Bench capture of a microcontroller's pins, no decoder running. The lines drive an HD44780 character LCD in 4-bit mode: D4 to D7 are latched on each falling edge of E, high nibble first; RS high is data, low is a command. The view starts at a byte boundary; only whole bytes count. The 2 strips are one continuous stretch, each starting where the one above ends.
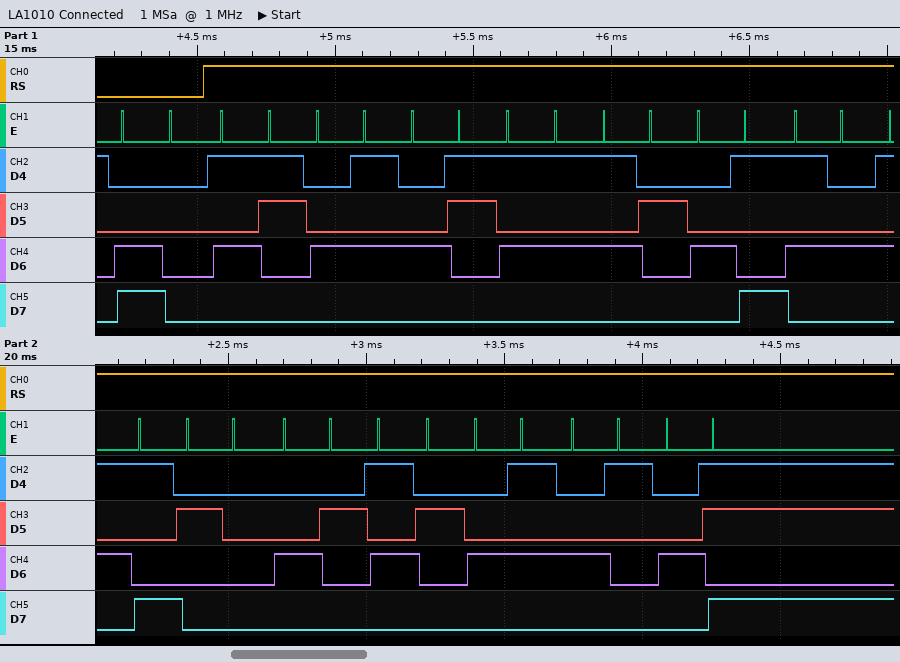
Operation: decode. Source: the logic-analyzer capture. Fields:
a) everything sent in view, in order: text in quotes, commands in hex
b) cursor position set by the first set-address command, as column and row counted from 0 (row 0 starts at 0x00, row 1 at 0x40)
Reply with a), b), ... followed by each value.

a) 0xC0 "SECURITY BREAK"
b) column 0, row 1
